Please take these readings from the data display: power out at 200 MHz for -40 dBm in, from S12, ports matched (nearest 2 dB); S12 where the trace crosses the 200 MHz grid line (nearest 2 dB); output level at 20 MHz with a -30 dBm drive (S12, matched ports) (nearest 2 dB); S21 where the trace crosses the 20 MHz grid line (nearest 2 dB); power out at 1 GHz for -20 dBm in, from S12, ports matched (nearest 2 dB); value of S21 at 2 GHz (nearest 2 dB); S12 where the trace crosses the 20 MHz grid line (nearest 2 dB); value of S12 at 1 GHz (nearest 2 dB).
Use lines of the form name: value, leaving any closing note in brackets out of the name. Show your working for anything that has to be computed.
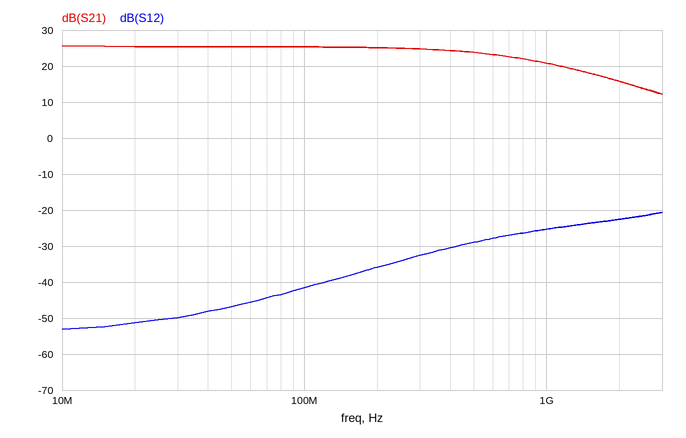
power out at 200 MHz for -40 dBm in, from S12, ports matched: -40 dBm + (-36 dB) = -76 dBm
S12 where the trace crosses the 200 MHz grid line: -36 dB
output level at 20 MHz with a -30 dBm drive (S12, matched ports): -30 dBm + (-52 dB) = -82 dBm
S21 where the trace crosses the 20 MHz grid line: 26 dB
power out at 1 GHz for -20 dBm in, from S12, ports matched: -20 dBm + (-26 dB) = -46 dBm
value of S21 at 2 GHz: 16 dB
S12 where the trace crosses the 20 MHz grid line: -52 dB
value of S12 at 1 GHz: -26 dB
